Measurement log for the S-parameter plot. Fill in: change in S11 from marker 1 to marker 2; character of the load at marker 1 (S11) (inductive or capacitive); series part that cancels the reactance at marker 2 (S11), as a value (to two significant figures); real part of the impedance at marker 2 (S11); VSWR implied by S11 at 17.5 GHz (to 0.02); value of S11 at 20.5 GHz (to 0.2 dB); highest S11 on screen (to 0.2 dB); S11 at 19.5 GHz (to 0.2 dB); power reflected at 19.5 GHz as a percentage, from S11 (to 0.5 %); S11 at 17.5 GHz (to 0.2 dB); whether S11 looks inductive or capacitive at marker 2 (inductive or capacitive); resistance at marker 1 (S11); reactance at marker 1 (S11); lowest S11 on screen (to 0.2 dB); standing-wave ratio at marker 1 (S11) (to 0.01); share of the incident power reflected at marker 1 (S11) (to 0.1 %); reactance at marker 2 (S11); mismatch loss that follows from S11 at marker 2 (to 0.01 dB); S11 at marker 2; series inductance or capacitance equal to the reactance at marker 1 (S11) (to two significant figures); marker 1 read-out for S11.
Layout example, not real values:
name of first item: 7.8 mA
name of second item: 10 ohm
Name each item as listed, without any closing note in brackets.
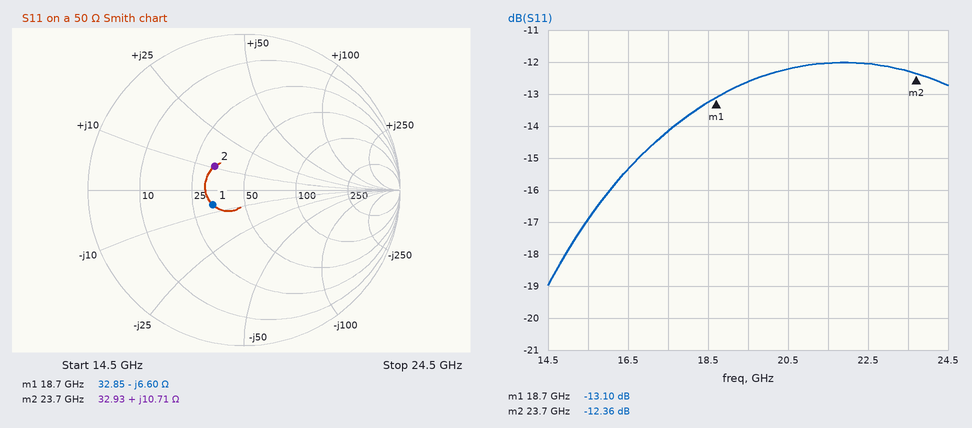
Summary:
change in S11 from marker 1 to marker 2: 0.74 dB
character of the load at marker 1 (S11): capacitive
series part that cancels the reactance at marker 2 (S11), as a value: 630 fF
real part of the impedance at marker 2: 32.93 Ω
VSWR implied by S11 at 17.5 GHz: 1.48
value of S11 at 20.5 GHz: -12.2 dB
highest S11 on screen: -12.0 dB
S11 at 19.5 GHz: -12.6 dB
power reflected at 19.5 GHz as a percentage, from S11: 5.5 %
S11 at 17.5 GHz: -14.2 dB
whether S11 looks inductive or capacitive at marker 2: inductive
resistance at marker 1: 32.85 Ω
reactance at marker 1: -6.60 Ω
lowest S11 on screen: -19.0 dB
standing-wave ratio at marker 1 (S11): 1.57
share of the incident power reflected at marker 1 (S11): 4.9 %
reactance at marker 2: +10.71 Ω
mismatch loss that follows from S11 at marker 2: 0.26 dB
S11 at marker 2: -12.36 dB
series inductance or capacitance equal to the reactance at marker 1 (S11): 1.3 pF
marker 1 read-out for S11: -13.10 dB
